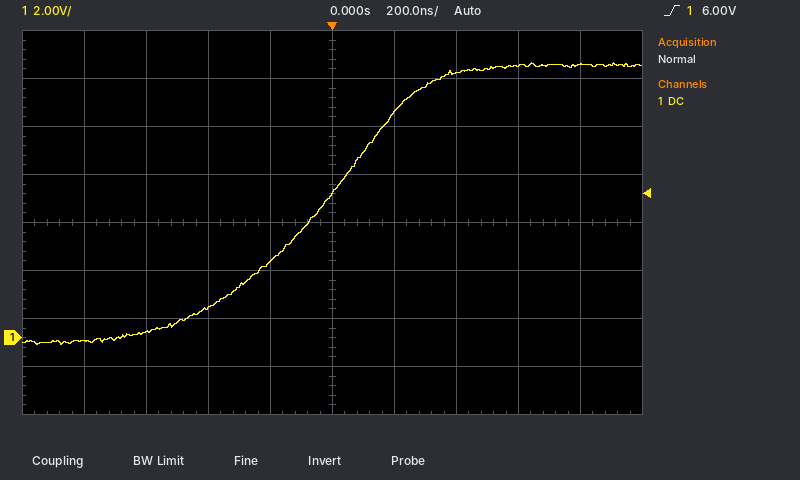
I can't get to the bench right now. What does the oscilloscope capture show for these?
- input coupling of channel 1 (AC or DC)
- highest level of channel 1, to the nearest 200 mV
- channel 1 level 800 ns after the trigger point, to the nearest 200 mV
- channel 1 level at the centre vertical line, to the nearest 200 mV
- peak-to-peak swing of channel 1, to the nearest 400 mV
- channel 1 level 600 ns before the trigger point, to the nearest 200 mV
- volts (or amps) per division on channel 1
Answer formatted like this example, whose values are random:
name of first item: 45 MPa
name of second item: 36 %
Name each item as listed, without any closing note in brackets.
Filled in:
input coupling of channel 1: DC
highest level of channel 1, to the nearest 200 mV: 11.4 V
channel 1 level 800 ns after the trigger point, to the nearest 200 mV: 11.4 V
channel 1 level at the centre vertical line, to the nearest 200 mV: 6.0 V
peak-to-peak swing of channel 1, to the nearest 400 mV: 11.6 V
channel 1 level 600 ns before the trigger point, to the nearest 200 mV: 200 mV
volts (or amps) per division on channel 1: 2 V
